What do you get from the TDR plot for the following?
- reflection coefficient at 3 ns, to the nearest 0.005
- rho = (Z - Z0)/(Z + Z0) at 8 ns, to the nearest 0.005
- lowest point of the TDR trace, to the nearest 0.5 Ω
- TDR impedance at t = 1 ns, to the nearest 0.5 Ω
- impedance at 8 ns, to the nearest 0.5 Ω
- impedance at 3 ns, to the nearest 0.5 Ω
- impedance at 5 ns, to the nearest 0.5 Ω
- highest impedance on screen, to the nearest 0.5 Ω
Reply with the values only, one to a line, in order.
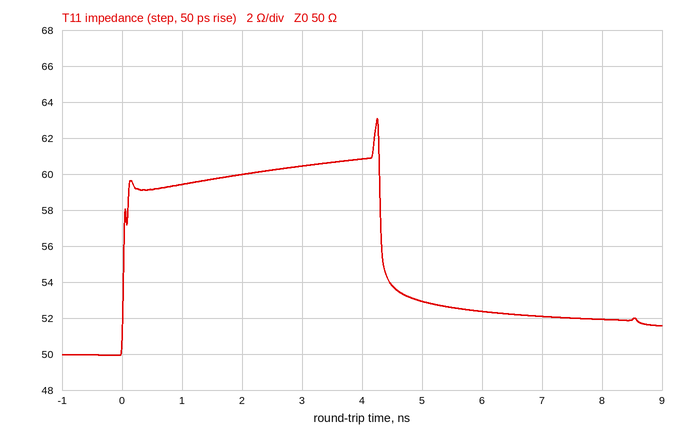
+0.095
+0.020
50.0 Ω
59.5 Ω
52.0 Ω
60.5 Ω
53.0 Ω
63.0 Ω
